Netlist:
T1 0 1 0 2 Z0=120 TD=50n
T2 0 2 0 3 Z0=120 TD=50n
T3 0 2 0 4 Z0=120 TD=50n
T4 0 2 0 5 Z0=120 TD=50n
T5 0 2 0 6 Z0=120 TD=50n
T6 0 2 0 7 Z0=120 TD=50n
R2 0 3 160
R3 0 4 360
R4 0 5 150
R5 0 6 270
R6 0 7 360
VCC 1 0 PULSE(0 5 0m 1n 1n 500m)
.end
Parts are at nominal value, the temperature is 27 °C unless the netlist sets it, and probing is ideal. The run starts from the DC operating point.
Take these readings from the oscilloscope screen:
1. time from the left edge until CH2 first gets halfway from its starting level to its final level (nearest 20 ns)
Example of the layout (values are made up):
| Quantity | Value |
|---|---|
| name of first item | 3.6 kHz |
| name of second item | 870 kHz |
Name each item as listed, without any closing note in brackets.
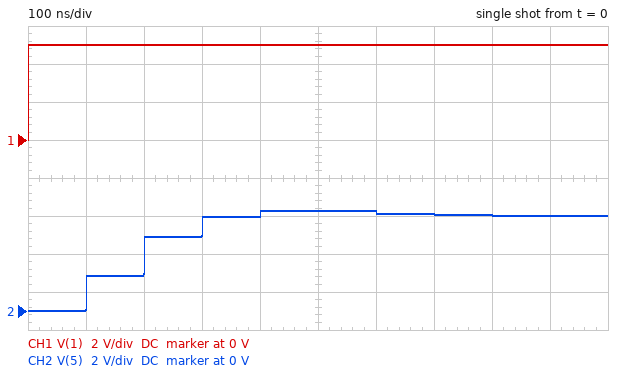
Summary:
| Quantity | Value |
|---|---|
| time from the left edge until CH2 first gets halfway from its starting level to its final level | 200 ns |
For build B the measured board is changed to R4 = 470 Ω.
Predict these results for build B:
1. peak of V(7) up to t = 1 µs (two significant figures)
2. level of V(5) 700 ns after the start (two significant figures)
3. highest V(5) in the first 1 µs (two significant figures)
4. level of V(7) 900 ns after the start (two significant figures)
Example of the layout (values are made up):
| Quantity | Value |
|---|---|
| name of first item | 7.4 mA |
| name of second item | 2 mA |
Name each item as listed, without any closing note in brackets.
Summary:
| Quantity | Value |
|---|---|
| peak of V(7) up to t = 1 µs | 5.8 V |
| level of V(5) 700 ns after the start | 5.1 V |
| highest V(5) in the first 1 µs | 5.7 V |
| level of V(7) 900 ns after the start | 4.9 V |
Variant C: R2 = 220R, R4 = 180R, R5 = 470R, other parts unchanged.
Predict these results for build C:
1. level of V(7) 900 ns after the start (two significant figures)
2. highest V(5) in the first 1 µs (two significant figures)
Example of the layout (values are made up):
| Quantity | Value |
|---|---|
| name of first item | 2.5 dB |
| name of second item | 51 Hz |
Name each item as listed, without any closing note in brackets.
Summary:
| Quantity | Value |
|---|---|
| level of V(7) 900 ns after the start | 4.9 V |
| highest V(5) in the first 1 µs | 5.8 V |
